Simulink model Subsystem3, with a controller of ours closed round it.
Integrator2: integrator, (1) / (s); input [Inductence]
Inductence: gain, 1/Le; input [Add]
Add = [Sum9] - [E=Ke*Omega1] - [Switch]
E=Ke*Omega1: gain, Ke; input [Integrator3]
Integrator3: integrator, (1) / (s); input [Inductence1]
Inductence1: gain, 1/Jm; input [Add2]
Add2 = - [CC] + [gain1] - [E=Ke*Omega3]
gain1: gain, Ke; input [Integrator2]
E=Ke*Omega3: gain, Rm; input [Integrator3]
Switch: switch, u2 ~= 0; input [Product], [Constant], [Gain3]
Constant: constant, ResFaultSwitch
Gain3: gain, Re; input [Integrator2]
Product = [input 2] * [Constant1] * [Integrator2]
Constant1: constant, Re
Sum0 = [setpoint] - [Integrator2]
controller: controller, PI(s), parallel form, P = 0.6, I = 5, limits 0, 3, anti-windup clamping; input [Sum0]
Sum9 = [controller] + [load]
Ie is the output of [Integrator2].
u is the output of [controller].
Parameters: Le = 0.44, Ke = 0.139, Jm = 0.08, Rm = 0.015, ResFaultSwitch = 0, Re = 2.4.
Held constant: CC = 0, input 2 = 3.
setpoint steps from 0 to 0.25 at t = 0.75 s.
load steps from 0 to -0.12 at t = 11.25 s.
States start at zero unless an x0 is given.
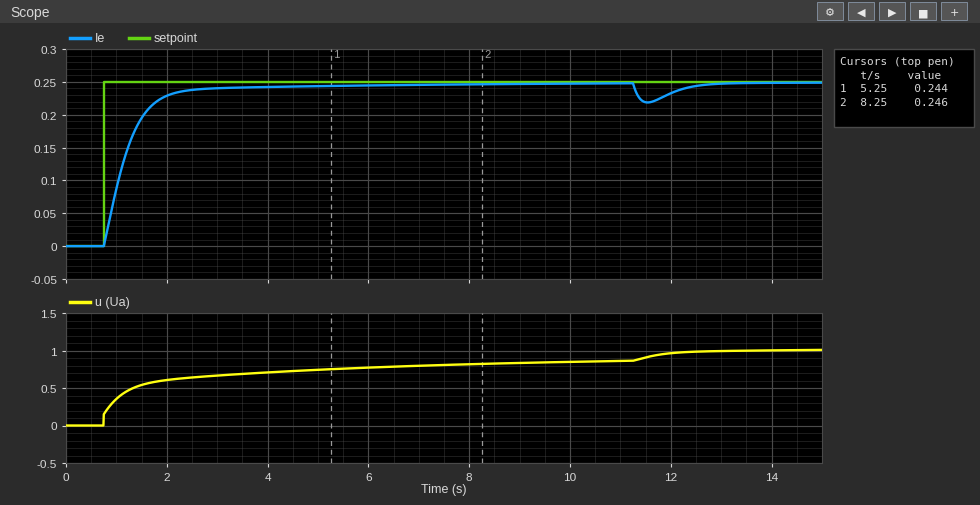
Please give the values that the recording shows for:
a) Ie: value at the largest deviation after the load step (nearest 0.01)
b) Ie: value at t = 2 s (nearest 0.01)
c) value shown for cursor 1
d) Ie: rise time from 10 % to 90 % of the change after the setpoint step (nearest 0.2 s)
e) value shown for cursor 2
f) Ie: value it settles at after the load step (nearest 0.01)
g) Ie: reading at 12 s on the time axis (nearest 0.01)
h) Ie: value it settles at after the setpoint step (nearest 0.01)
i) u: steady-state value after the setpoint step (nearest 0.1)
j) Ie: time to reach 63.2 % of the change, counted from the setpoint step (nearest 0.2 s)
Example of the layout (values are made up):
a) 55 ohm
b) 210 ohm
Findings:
a) 0.22
b) 0.23
c) 0.244
d) 1.0 s
e) 0.246
f) 0.25
g) 0.23
h) 0.25
i) 0.9
j) 0.6 s
